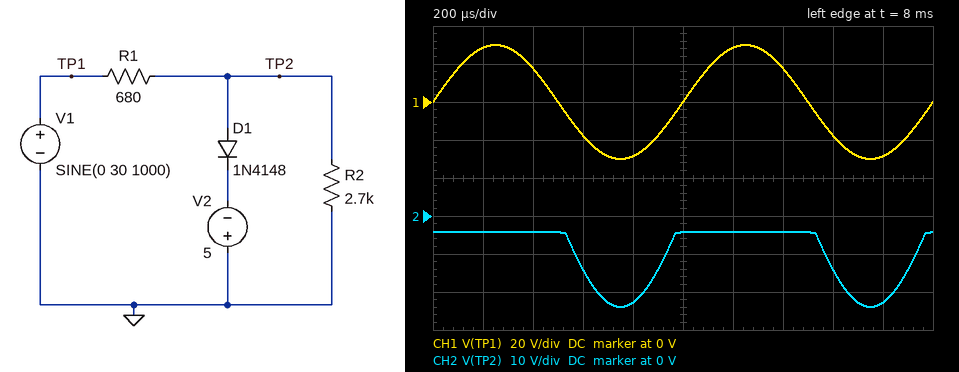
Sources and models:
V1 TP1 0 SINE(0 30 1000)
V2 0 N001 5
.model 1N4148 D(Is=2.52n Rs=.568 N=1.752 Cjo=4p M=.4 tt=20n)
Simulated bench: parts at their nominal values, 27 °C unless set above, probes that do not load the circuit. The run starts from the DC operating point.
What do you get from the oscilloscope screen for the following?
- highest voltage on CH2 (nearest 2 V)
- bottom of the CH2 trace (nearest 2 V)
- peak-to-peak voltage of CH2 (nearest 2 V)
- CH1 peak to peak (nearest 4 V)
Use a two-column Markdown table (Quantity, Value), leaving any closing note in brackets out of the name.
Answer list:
| Quantity | Value |
|---|---|
| highest voltage on CH2 | -4 V |
| bottom of the CH2 trace | -24 V |
| peak-to-peak voltage of CH2 | 20 V |
| CH1 peak to peak | 60 V |
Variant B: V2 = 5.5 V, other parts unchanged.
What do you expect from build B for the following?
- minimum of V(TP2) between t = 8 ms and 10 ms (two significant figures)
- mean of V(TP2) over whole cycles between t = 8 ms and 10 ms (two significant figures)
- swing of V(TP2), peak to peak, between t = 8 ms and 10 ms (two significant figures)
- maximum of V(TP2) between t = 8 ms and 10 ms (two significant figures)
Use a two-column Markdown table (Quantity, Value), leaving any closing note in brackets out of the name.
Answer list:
| Quantity | Value |
|---|---|
| minimum of V(TP2) between t = 8 ms and 10 ms | -24 V |
| mean of V(TP2) over whole cycles between t = 8 ms and 10 ms | -10 V |
| swing of V(TP2), peak to peak, between t = 8 ms and 10 ms | 19 V |
| maximum of V(TP2) between t = 8 ms and 10 ms | -4.7 V |
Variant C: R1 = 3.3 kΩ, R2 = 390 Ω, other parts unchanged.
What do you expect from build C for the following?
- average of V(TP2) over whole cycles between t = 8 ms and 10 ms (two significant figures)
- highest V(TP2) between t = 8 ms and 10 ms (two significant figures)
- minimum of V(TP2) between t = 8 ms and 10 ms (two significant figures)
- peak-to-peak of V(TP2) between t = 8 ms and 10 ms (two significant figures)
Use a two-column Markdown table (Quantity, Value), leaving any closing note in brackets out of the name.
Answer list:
| Quantity | Value |
|---|---|
| average of V(TP2) over whole cycles between t = 8 ms and 10 ms | -4.3 V |
| highest V(TP2) between t = 8 ms and 10 ms | -4.3 V |
| minimum of V(TP2) between t = 8 ms and 10 ms | -4.4 V |
| peak-to-peak of V(TP2) between t = 8 ms and 10 ms | 93 mV |
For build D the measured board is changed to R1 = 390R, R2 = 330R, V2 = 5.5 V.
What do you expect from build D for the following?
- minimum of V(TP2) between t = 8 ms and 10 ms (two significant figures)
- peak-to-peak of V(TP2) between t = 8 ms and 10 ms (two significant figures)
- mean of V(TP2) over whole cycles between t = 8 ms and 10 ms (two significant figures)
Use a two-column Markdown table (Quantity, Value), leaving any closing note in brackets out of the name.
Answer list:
| Quantity | Value |
|---|---|
| minimum of V(TP2) between t = 8 ms and 10 ms | -14 V |
| peak-to-peak of V(TP2) between t = 8 ms and 10 ms | 9.1 V |
| mean of V(TP2) over whole cycles between t = 8 ms and 10 ms | -7.0 V |
